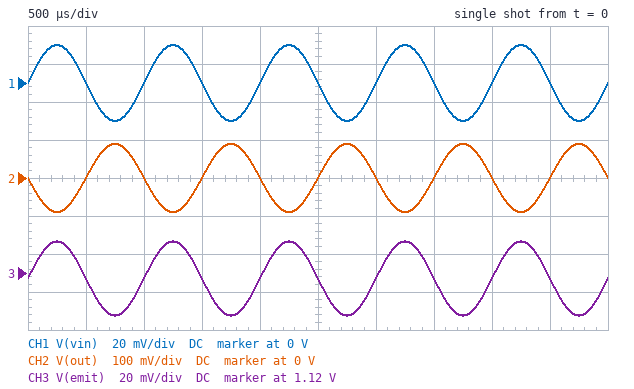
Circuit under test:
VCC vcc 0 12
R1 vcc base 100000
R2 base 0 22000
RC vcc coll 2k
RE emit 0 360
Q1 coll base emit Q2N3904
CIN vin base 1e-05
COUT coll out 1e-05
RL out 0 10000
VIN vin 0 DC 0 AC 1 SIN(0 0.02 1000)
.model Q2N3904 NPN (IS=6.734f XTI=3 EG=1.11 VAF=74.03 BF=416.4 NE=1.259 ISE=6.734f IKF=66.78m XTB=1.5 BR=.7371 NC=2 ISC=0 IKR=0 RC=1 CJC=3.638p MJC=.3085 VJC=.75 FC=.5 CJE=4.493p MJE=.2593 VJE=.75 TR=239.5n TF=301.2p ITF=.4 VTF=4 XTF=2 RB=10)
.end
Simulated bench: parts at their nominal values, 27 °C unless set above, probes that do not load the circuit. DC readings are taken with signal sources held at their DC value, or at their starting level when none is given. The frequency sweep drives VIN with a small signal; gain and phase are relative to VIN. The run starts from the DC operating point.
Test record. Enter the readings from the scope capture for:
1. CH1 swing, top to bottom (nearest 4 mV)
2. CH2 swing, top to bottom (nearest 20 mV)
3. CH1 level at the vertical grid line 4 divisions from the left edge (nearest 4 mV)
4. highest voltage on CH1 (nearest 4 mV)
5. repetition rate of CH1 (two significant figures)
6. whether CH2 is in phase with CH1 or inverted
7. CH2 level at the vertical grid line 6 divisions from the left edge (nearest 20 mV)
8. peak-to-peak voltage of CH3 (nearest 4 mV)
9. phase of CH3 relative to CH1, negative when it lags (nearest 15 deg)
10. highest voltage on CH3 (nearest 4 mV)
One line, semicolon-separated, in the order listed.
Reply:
40 mV; 180 mV; 0 V; 20 mV; 1.0 kHz; inverted; 0 V; 40 mV; 0 deg; 1.136 V
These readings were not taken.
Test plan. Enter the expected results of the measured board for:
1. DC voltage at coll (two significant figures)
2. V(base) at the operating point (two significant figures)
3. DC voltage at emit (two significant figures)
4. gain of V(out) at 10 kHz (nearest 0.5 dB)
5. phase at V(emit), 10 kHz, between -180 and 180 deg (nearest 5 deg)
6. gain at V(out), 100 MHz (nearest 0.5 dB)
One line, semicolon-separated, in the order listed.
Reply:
5.8 V; 1.8 V; 1.1 V; 13.0 dB; 0 deg; 6.5 dB
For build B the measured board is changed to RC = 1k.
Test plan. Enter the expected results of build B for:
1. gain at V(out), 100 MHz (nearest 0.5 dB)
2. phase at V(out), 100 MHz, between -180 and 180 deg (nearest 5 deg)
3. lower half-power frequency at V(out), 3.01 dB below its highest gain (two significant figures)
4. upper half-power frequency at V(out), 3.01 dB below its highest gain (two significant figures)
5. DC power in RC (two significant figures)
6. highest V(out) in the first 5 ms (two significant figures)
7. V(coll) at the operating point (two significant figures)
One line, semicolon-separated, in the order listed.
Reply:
5.5 dB; 100 deg; 2.0 Hz; 140 MHz; 9.7 mW; 49 mV; 8.9 V
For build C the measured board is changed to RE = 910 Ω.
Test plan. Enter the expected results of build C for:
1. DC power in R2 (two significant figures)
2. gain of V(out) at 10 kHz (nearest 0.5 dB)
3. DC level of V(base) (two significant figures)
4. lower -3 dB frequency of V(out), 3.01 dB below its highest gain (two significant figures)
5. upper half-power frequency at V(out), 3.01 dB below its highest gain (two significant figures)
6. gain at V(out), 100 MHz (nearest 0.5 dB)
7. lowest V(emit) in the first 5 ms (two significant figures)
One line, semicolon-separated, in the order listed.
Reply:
180 µW; 5.0 dB; 2.0 V; 1.8 Hz; 130 MHz; 2.5 dB; 1.3 V
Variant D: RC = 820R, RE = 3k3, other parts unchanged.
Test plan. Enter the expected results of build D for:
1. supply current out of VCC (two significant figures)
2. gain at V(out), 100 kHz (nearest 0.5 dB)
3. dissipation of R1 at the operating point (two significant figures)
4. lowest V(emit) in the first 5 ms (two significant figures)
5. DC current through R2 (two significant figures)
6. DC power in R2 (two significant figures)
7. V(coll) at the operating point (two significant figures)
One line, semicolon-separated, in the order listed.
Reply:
540 µA; -13.0 dB; 980 µW; 1.4 V; 96 µA; 200 µW; 12 V
